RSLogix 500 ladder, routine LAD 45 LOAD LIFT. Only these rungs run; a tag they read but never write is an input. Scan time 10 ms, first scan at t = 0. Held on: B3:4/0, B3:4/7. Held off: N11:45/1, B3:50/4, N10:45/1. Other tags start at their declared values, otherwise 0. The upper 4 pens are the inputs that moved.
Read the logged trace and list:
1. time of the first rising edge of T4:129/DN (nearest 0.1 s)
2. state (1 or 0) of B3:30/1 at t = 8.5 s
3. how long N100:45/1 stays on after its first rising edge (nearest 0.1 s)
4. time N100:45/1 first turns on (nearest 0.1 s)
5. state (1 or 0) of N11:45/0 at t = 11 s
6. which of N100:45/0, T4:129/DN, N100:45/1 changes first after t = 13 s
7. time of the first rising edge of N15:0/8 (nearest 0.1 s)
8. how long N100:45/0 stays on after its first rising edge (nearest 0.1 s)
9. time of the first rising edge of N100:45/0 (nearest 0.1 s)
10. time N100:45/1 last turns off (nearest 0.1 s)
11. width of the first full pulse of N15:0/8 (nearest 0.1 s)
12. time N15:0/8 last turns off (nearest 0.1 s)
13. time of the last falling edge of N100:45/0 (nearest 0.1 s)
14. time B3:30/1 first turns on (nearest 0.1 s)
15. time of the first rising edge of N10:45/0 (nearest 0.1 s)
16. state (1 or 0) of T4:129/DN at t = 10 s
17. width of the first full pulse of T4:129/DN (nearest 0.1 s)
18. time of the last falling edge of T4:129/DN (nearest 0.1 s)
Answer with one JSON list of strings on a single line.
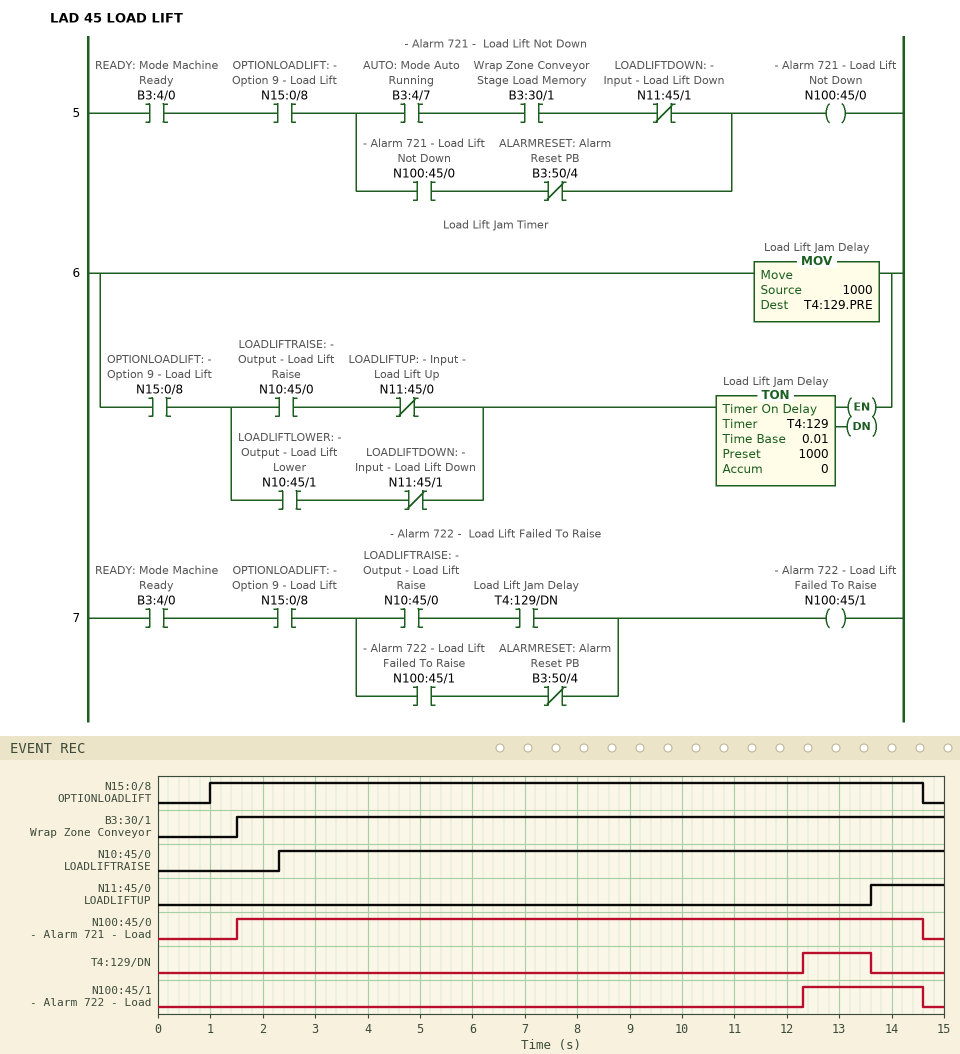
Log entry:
["12.3 s", "1", "2.3 s", "12.3 s", "0", "T4:129/DN", "1.0 s", "13.1 s", "1.5 s", "14.6 s", "13.6 s", "14.6 s", "14.6 s", "1.5 s", "2.3 s", "0", "1.3 s", "13.6 s"]
